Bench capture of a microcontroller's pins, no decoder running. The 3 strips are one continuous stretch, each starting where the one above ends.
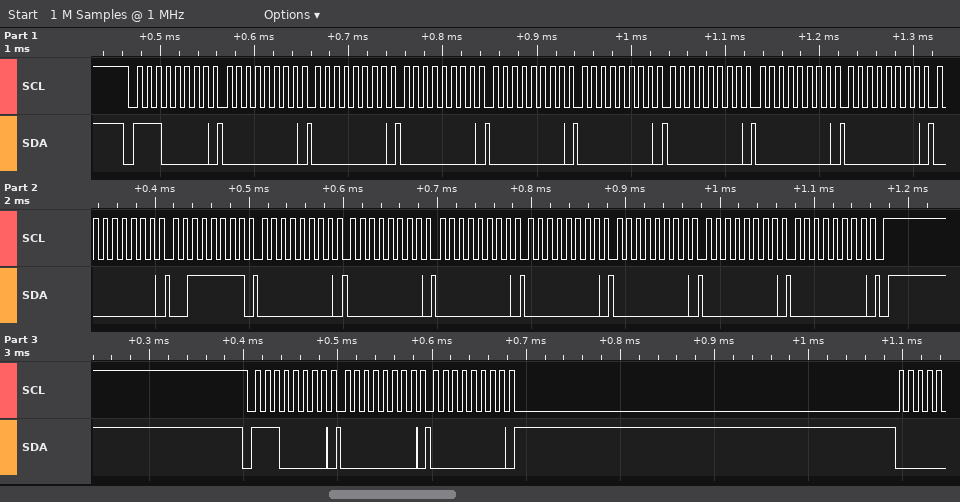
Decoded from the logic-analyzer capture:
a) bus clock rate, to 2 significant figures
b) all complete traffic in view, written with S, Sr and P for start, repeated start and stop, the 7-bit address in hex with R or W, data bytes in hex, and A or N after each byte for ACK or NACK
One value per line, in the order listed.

100 kHz
S 70W A 00 A 00 A 00 A 00 A 00 A 00 A 00 A 00 A 00 A 3F A 00 A 00 A 00 A 00 A 00 A 00 A 00 A P S 70W A 00 A 00 A
